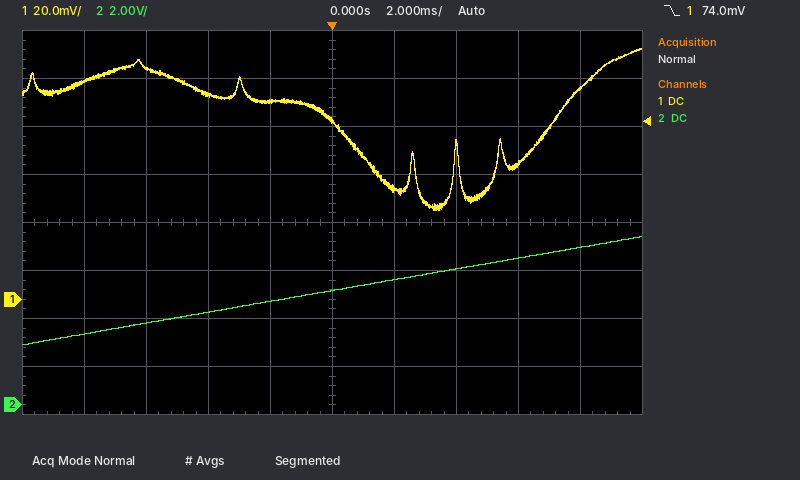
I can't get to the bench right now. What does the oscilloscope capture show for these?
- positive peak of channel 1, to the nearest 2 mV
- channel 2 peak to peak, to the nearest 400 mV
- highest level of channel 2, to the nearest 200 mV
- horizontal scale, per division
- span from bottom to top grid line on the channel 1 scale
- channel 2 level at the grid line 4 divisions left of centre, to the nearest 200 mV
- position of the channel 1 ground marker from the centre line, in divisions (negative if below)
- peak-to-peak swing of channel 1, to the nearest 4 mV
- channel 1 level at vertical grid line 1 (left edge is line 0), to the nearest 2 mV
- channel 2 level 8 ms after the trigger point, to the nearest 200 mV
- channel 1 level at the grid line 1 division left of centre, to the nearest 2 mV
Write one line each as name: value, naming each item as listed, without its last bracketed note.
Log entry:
positive peak of channel 1, to the nearest 2 mV: 104 mV
channel 2 peak to peak, to the nearest 400 mV: 4.4 V
highest level of channel 2, to the nearest 200 mV: 7.0 V
horizontal scale, per division: 2 ms
span from bottom to top grid line on the channel 1 scale: 160 mV
channel 2 level at the grid line 4 divisions left of centre, to the nearest 200 mV: 3.0 V
position of the channel 1 ground marker from the centre line, in divisions: -1.6 div
peak-to-peak swing of channel 1, to the nearest 4 mV: 68 mV
channel 1 level at vertical grid line 1 (left edge is line 0), to the nearest 2 mV: 90 mV
channel 2 level 8 ms after the trigger point, to the nearest 200 mV: 6.6 V
channel 1 level at the grid line 1 division left of centre, to the nearest 2 mV: 82 mV
